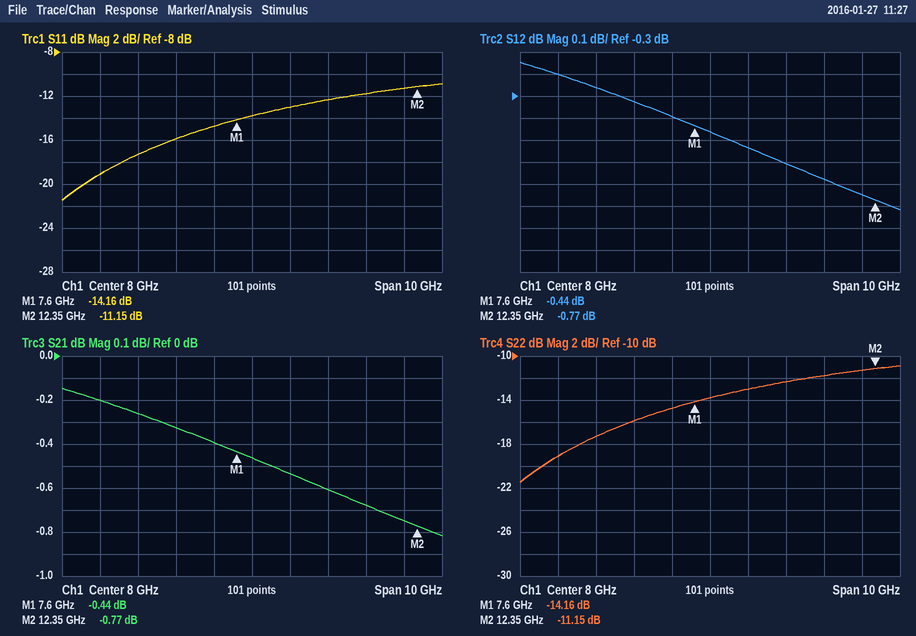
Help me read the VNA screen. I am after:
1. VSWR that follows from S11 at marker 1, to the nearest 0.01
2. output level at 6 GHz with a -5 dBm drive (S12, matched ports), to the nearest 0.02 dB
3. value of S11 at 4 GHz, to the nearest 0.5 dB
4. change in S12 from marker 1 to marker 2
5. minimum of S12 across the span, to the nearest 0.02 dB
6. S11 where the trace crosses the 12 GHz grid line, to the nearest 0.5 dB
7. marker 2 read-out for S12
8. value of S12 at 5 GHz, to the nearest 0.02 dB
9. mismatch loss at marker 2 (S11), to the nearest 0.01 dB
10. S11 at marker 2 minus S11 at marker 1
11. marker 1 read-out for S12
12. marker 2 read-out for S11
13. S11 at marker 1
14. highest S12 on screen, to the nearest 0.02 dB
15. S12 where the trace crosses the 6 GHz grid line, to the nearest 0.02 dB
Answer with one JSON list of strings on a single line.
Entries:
["1.49", "-5.32 dBm", "-19.0 dB", "-0.33 dB", "-0.82 dB", "-11.5 dB", "-0.77 dB", "-0.26 dB", "0.35 dB", "3.01 dB", "-0.44 dB", "-11.15 dB", "-14.16 dB", "-0.14 dB", "-0.32 dB"]
